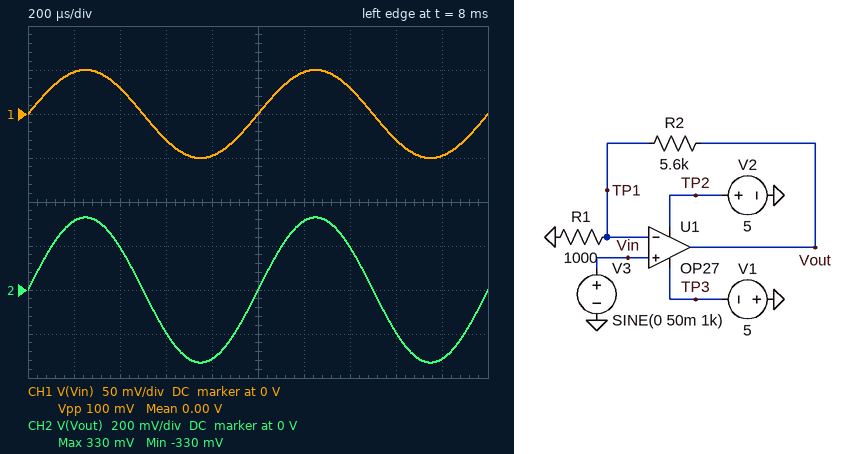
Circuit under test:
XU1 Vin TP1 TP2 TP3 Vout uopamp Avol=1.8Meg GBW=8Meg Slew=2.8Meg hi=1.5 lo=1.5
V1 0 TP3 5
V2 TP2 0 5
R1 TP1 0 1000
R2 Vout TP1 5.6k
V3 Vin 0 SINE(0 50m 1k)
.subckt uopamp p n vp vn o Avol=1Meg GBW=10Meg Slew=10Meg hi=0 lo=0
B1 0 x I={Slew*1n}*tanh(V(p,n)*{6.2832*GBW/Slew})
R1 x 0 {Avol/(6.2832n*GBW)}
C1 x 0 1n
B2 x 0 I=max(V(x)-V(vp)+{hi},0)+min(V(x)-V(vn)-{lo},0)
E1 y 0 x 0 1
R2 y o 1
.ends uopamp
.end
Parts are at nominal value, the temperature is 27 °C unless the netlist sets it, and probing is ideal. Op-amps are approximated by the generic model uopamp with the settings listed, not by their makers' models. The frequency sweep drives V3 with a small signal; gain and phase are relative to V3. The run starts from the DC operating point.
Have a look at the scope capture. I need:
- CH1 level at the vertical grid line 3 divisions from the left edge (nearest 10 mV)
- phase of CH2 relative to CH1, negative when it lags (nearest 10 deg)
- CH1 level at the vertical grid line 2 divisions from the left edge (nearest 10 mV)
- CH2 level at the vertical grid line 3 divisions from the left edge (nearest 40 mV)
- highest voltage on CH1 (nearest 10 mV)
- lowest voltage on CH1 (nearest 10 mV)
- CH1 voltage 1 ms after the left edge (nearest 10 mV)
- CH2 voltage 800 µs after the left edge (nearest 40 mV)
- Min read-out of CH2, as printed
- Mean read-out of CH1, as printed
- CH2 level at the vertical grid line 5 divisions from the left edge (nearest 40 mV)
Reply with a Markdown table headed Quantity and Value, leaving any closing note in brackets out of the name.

| Quantity | Value |
|---|---|
| CH1 level at the vertical grid line 3 divisions from the left edge | -30 mV |
| phase of CH2 relative to CH1, negative when it lags | 0 deg |
| CH1 level at the vertical grid line 2 divisions from the left edge | 30 mV |
| CH2 level at the vertical grid line 3 divisions from the left edge | -200 mV |
| highest voltage on CH1 | 50 mV |
| lowest voltage on CH1 | -50 mV |
| CH1 voltage 1 ms after the left edge | 0 V |
| CH2 voltage 800 µs after the left edge | -320 mV |
| Min read-out of CH2, as printed | -330 mV |
| Mean read-out of CH1, as printed | 0.00 V |
| CH2 level at the vertical grid line 5 divisions from the left edge | 0 V |
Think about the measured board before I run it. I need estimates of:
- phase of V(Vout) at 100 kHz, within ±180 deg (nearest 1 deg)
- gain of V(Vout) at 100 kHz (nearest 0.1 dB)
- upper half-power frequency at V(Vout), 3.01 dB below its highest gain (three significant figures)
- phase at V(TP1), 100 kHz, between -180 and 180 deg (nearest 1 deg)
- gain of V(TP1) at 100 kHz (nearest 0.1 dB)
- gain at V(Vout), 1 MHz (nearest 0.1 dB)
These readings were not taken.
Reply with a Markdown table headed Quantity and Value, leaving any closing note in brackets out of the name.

| Quantity | Value |
|---|---|
| phase of V(Vout) at 100 kHz, within ±180 deg | -5 deg |
| gain of V(Vout) at 100 kHz | 16.4 dB |
| upper half-power frequency at V(Vout), 3.01 dB below its highest gain | 1.21 MHz |
| phase at V(TP1), 100 kHz, between -180 and 180 deg | -5 deg |
| gain of V(TP1) at 100 kHz | 0 dB |
| gain at V(Vout), 1 MHz | 14.1 dB |
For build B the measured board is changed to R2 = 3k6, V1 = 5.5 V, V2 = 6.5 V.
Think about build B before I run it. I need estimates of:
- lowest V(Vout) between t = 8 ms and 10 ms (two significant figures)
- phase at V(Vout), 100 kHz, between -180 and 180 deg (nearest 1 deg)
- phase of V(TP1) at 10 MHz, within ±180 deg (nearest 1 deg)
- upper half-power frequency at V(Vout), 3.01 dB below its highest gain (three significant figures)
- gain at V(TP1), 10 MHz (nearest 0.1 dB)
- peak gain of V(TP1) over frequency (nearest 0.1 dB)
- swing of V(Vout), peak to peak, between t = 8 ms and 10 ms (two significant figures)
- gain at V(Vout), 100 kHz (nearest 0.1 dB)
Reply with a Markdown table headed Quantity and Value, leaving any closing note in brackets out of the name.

| Quantity | Value |
|---|---|
| lowest V(Vout) between t = 8 ms and 10 ms | -230 mV |
| phase at V(Vout), 100 kHz, between -180 and 180 deg | -3 deg |
| phase of V(TP1) at 10 MHz, within ±180 deg | -80 deg |
| upper half-power frequency at V(Vout), 3.01 dB below its highest gain | 1.74 MHz |
| gain at V(TP1), 10 MHz | -15.3 dB |
| peak gain of V(TP1) over frequency | 0 dB |
| swing of V(Vout), peak to peak, between t = 8 ms and 10 ms | 460 mV |
| gain at V(Vout), 100 kHz | 13.2 dB |
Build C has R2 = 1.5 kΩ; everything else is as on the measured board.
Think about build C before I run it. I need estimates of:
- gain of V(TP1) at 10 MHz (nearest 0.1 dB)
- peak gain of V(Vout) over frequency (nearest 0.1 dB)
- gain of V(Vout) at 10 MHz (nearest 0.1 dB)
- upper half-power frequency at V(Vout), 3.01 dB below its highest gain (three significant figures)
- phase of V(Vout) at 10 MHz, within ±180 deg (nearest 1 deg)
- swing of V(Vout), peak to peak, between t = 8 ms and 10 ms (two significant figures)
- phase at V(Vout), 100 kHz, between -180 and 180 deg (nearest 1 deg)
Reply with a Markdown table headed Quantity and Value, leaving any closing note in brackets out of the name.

| Quantity | Value |
|---|---|
| gain of V(TP1) at 10 MHz | -10.3 dB |
| peak gain of V(Vout) over frequency | 8.0 dB |
| gain of V(Vout) at 10 MHz | -2.4 dB |
| upper half-power frequency at V(Vout), 3.01 dB below its highest gain | 3.20 MHz |
| phase of V(Vout) at 10 MHz, within ±180 deg | -72 deg |
| swing of V(Vout), peak to peak, between t = 8 ms and 10 ms | 250 mV |
| phase at V(Vout), 100 kHz, between -180 and 180 deg | -2 deg |
